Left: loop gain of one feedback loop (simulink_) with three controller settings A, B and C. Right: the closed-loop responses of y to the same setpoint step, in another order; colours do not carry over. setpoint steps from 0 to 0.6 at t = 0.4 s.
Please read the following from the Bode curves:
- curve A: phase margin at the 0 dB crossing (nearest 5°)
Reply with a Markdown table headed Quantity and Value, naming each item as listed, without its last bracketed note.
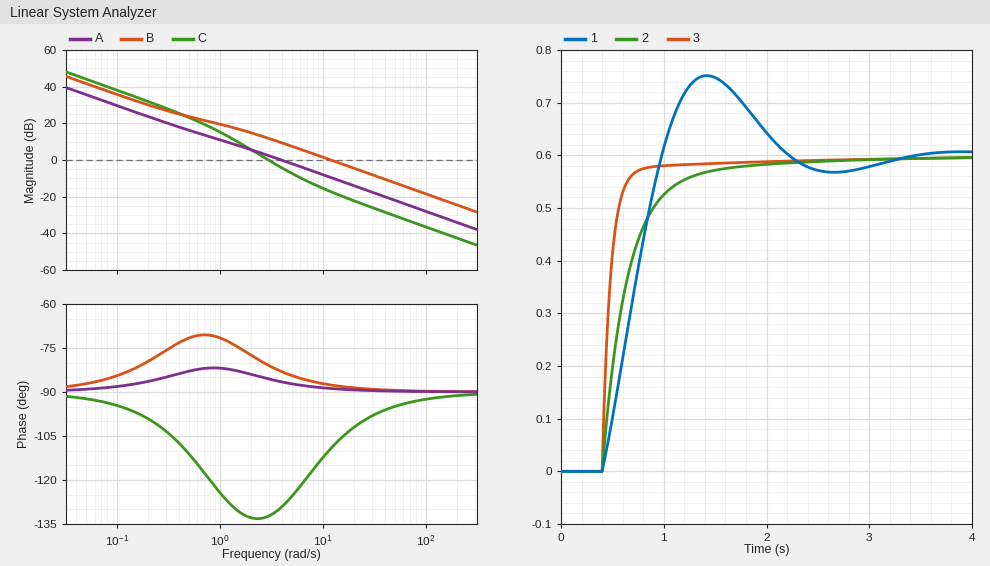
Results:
| Quantity | Value |
|---|---|
| curve A: phase margin at the 0 dB crossing | 95° |
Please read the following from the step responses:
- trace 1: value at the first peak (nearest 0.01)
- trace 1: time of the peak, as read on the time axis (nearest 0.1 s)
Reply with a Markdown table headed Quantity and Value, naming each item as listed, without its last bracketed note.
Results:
| Quantity | Value |
|---|---|
| trace 1: value at the first peak | 0.75 |
| trace 1: time of the peak, as read on the time axis | 1.4 s |
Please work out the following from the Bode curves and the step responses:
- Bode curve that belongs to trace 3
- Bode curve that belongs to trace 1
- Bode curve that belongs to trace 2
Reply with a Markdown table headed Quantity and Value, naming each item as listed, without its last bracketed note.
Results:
| Quantity | Value |
|---|---|
| Bode curve that belongs to trace 3 | B |
| Bode curve that belongs to trace 1 | C |
| Bode curve that belongs to trace 2 | A |
